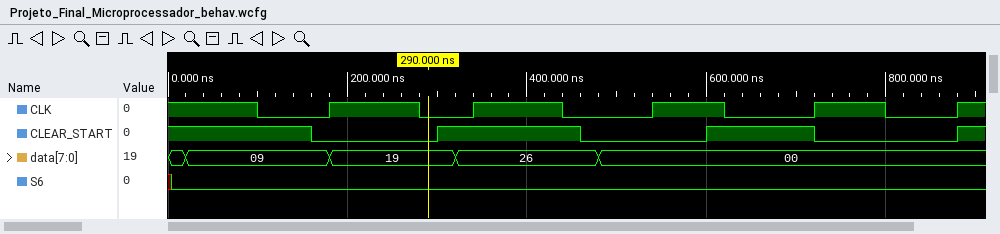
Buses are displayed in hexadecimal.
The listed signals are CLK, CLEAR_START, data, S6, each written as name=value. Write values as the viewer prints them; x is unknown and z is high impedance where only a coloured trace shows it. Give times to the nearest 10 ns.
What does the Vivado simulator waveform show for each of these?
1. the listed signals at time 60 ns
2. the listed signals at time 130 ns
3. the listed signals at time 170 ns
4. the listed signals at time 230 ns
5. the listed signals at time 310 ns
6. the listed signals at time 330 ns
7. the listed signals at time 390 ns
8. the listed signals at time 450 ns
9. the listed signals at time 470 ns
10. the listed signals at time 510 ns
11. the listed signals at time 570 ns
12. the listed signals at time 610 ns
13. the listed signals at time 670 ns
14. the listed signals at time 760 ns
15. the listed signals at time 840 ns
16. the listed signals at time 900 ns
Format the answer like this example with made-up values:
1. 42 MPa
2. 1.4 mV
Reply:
1. CLK=1, CLEAR_START=1, data=09, S6=0
2. CLK=0, CLEAR_START=1, data=09, S6=0
3. CLK=0, CLEAR_START=0, data=09, S6=0
4. CLK=1, CLEAR_START=0, data=19, S6=0
5. CLK=0, CLEAR_START=1, data=19, S6=0
6. CLK=0, CLEAR_START=1, data=26, S6=0
7. CLK=1, CLEAR_START=1, data=26, S6=0
8. CLK=0, CLEAR_START=1, data=26, S6=0
9. CLK=0, CLEAR_START=0, data=26, S6=0
10. CLK=0, CLEAR_START=0, data=00, S6=0
11. CLK=1, CLEAR_START=0, data=00, S6=0
12. CLK=1, CLEAR_START=1, data=00, S6=0
13. CLK=0, CLEAR_START=1, data=00, S6=0
14. CLK=1, CLEAR_START=0, data=00, S6=0
15. CLK=0, CLEAR_START=0, data=00, S6=0
16. CLK=1, CLEAR_START=1, data=00, S6=0
